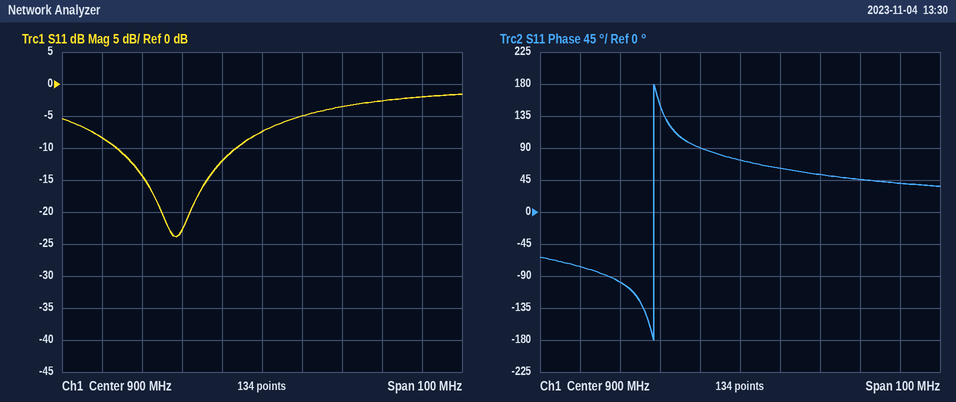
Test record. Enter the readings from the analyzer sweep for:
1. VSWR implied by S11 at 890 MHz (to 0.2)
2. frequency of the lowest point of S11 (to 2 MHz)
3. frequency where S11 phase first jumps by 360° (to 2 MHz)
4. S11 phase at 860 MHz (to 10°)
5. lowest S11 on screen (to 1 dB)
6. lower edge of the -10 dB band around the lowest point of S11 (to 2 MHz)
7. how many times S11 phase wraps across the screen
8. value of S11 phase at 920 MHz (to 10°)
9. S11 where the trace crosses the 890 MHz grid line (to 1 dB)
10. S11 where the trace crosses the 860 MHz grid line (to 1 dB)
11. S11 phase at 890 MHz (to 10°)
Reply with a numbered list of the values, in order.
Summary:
1. 1.6
2. 878 MHz
3. 878 MHz
4. -80°
5. -24 dB
6. 864 MHz
7. 1
8. 50°
9. -12 dB
10. -8 dB
11. 90°
